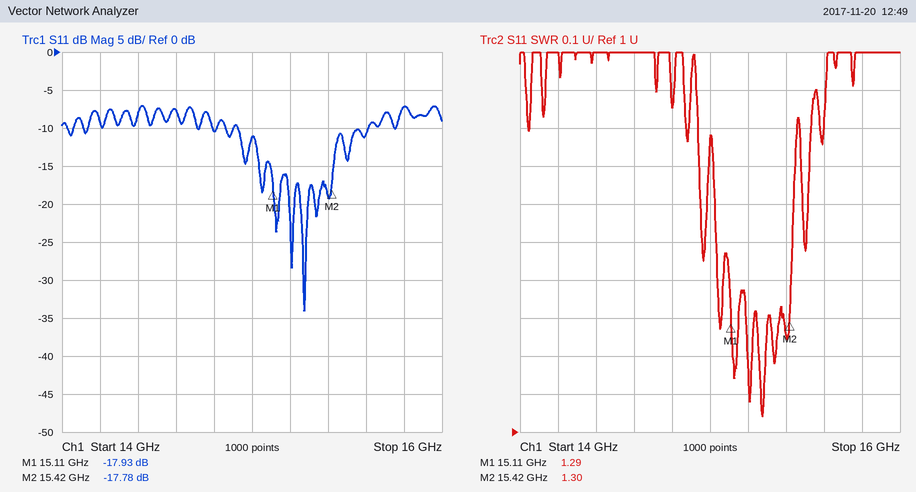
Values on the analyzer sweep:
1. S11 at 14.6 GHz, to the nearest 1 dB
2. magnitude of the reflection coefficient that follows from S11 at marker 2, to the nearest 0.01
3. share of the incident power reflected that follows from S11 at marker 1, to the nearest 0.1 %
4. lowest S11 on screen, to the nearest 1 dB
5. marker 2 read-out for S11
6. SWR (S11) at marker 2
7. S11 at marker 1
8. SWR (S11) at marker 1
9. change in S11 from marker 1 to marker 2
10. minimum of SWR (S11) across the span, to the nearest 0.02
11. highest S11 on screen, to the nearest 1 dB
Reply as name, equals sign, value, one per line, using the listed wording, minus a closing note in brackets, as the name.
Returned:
S11 at 14.6 GHz, to the nearest 1 dB = -8 dB
magnitude of the reflection coefficient that follows from S11 at marker 2, to the nearest 0.01 = 0.13
share of the incident power reflected that follows from S11 at marker 1, to the nearest 0.1 % = 1.6 %
lowest S11 on screen, to the nearest 1 dB = -34 dB
marker 2 read-out for S11 = -17.78 dB
SWR (S11) at marker 2 = 1.30
S11 at marker 1 = -17.93 dB
SWR (S11) at marker 1 = 1.29
change in S11 from marker 1 to marker 2 = 0.15 dB
minimum of SWR (S11) across the span, to the nearest 0.02 = 1.04
highest S11 on screen, to the nearest 1 dB = -7 dB
